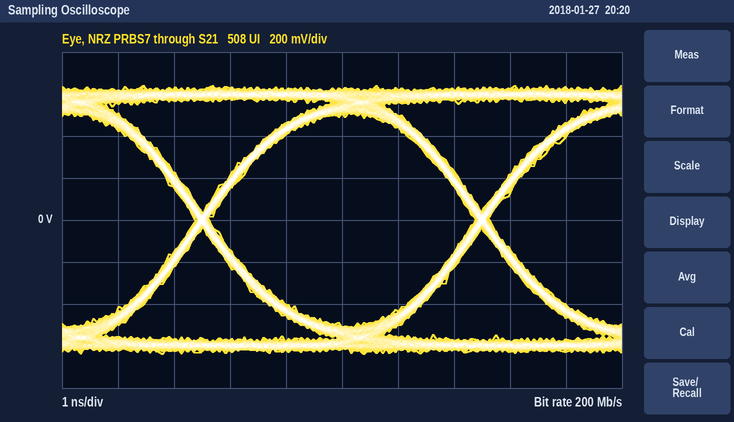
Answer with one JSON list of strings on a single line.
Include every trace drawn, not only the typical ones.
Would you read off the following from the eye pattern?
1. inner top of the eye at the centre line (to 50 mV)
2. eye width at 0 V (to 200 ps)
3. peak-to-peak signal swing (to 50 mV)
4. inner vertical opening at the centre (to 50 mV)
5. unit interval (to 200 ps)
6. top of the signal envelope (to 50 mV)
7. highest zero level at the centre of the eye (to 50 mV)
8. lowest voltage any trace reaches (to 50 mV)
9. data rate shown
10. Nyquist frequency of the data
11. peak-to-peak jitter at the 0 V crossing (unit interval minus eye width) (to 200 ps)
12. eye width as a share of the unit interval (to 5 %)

["500 mV", "4.8 ns", "1.30 V", "1.00 V", "5.0 ns", "650 mV", "-500 mV", "-650 mV", "200 Mb/s", "100 MHz", "200 ps", "95 %"]
